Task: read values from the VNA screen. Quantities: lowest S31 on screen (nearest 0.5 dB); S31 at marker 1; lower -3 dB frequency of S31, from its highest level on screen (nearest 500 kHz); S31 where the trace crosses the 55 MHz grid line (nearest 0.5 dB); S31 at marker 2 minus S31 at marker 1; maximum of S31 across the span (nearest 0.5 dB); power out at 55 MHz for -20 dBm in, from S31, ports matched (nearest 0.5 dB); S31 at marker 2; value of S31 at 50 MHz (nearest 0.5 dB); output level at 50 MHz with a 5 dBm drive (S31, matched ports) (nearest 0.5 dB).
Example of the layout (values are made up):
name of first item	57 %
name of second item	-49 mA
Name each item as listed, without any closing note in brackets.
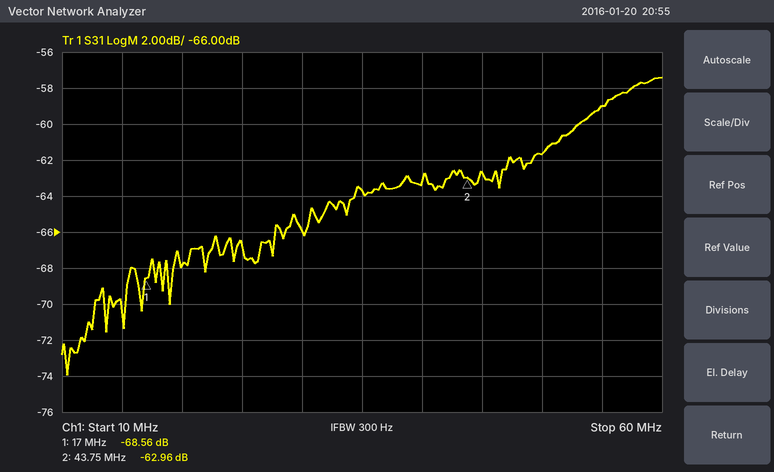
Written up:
lowest S31 on screen	-74.0 dB
S31 at marker 1	-68.56 dB
lower -3 dB frequency of S31, from its highest level on screen	52.5 MHz
S31 where the trace crosses the 55 MHz grid line	-59.0 dB
S31 at marker 2 minus S31 at marker 1	5.60 dB
maximum of S31 across the span	-57.5 dB
power out at 55 MHz for -20 dBm in, from S31, ports matched	-79.0 dBm
S31 at marker 2	-62.96 dB
value of S31 at 50 MHz	-61.5 dB
output level at 50 MHz with a 5 dBm drive (S31, matched ports)	-56.5 dBm
